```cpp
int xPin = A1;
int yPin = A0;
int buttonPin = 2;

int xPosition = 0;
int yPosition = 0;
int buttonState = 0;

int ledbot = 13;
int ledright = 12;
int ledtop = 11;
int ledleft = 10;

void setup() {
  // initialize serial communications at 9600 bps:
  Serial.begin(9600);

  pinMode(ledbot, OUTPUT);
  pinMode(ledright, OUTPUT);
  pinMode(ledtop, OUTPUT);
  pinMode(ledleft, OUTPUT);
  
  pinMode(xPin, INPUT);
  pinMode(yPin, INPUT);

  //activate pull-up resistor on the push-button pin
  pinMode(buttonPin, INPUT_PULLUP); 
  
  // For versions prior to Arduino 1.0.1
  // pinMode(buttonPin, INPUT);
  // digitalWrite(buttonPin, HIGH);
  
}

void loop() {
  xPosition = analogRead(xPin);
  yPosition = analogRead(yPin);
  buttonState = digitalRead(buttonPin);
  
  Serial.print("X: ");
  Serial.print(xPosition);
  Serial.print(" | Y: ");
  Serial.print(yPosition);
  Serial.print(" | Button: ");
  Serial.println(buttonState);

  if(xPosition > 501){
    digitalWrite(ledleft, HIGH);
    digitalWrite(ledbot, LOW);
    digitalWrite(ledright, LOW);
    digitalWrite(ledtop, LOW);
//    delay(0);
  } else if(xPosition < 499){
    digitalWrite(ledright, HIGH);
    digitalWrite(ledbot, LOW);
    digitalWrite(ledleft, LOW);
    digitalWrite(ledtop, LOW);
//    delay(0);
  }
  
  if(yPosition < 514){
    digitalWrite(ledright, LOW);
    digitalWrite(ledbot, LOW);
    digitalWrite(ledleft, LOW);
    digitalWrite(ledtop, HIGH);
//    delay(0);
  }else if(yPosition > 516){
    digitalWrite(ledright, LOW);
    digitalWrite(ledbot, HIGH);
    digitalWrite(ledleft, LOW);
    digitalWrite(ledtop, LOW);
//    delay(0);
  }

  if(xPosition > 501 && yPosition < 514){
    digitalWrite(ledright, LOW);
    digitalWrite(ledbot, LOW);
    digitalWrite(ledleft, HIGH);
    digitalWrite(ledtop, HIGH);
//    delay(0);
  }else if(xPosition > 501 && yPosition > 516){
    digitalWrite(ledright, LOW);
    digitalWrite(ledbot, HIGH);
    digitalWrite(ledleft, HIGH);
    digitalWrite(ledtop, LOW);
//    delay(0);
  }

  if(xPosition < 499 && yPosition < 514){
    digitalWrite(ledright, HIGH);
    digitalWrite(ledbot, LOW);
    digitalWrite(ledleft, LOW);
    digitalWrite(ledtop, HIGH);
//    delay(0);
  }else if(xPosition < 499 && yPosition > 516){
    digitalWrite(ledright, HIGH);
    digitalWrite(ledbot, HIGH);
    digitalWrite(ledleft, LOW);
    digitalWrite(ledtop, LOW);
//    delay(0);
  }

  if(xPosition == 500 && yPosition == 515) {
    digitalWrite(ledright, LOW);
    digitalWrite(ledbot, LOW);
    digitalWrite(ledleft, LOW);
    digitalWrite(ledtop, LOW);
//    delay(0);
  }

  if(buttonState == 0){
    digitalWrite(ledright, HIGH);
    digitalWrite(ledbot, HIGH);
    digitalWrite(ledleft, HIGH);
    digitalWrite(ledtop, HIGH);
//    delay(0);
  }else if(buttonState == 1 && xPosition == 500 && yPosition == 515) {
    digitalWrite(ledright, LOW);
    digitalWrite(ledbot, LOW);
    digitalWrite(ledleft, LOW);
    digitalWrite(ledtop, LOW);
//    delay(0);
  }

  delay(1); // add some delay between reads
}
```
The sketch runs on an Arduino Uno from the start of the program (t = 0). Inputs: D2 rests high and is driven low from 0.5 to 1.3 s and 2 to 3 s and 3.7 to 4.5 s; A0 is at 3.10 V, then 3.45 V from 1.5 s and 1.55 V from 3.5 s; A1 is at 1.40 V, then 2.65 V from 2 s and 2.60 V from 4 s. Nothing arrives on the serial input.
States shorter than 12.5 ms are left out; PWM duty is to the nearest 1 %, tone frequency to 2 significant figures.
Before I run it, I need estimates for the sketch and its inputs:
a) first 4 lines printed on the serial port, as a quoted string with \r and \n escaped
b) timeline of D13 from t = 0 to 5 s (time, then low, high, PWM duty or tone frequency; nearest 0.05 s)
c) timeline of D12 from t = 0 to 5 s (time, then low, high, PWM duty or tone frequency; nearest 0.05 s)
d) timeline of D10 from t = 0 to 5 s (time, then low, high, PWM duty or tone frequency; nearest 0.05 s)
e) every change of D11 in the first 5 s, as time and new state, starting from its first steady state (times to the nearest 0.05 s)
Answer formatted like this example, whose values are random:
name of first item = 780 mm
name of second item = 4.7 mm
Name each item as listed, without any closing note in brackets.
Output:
first 4 lines printed on the serial port, as a quoted string with \r and \n escaped = "X: 286 | Y: 634 | Button: 1\r\nX: 286 | Y: 634 | Button: 1\r\nX: 286 | Y: 634 | Button: 1\r\nX: 286 | Y: 634 | Button: 1\r\n"
timeline of D13 from t = 0 to 5 s = 0 s high; 3.55 s low; 3.75 s high; 4.55 s low
timeline of D12 from t = 0 to 5 s = 0 s high; 3.05 s low; 3.75 s high; 4.55 s low
timeline of D10 from t = 0 to 5 s = 0 s low; 0.55 s high; 1.35 s low; 2.05 s high
every change of D11 in the first 5 s, as time and new state, starting from its first steady state = 0 s low; 0.55 s high; 1.35 s low; 2.05 s high; 3.05 s low; 3.55 s high
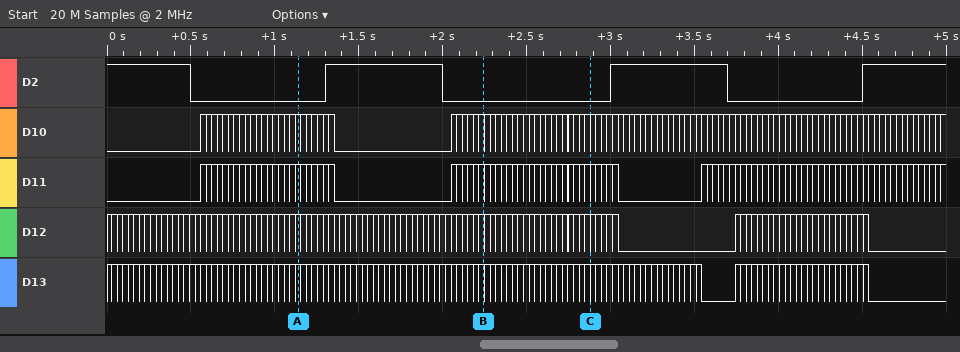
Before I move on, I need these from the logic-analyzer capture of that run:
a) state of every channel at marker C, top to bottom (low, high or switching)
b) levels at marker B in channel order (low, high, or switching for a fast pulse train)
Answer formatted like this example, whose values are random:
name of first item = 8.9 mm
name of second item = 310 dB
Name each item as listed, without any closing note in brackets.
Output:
state of every channel at marker C, top to bottom = D2 low, D10 high, D11 high, D12 high, D13 high
levels at marker B in channel order = D2 low, D10 high, D11 high, D12 high, D13 high
